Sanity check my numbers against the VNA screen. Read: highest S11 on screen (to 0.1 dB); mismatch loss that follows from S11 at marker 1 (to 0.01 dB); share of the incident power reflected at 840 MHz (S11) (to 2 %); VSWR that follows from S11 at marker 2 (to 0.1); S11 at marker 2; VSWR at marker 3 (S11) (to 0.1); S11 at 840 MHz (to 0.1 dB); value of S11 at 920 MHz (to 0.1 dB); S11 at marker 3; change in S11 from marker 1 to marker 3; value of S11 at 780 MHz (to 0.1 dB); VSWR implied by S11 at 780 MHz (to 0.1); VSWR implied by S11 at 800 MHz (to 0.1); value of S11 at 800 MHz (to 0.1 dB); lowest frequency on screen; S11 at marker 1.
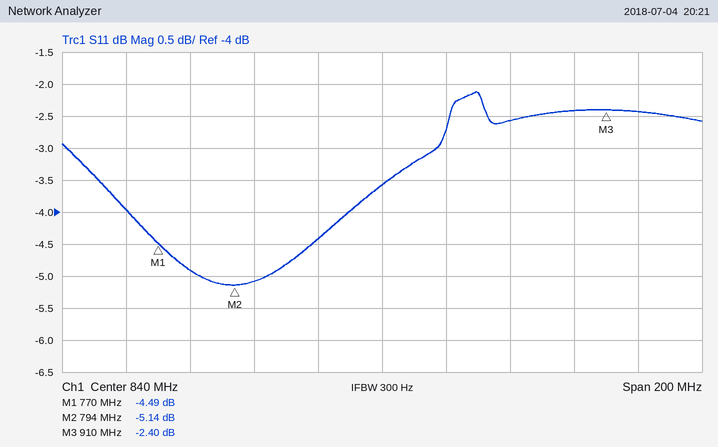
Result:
-2.1 dB
1.91 dB
44 %
3.5
-5.14 dB
7.3
-3.6 dB
-2.4 dB
-2.40 dB
2.09 dB
-4.9 dB
3.6
3.5
-5.1 dB
740 MHz
-4.49 dB
